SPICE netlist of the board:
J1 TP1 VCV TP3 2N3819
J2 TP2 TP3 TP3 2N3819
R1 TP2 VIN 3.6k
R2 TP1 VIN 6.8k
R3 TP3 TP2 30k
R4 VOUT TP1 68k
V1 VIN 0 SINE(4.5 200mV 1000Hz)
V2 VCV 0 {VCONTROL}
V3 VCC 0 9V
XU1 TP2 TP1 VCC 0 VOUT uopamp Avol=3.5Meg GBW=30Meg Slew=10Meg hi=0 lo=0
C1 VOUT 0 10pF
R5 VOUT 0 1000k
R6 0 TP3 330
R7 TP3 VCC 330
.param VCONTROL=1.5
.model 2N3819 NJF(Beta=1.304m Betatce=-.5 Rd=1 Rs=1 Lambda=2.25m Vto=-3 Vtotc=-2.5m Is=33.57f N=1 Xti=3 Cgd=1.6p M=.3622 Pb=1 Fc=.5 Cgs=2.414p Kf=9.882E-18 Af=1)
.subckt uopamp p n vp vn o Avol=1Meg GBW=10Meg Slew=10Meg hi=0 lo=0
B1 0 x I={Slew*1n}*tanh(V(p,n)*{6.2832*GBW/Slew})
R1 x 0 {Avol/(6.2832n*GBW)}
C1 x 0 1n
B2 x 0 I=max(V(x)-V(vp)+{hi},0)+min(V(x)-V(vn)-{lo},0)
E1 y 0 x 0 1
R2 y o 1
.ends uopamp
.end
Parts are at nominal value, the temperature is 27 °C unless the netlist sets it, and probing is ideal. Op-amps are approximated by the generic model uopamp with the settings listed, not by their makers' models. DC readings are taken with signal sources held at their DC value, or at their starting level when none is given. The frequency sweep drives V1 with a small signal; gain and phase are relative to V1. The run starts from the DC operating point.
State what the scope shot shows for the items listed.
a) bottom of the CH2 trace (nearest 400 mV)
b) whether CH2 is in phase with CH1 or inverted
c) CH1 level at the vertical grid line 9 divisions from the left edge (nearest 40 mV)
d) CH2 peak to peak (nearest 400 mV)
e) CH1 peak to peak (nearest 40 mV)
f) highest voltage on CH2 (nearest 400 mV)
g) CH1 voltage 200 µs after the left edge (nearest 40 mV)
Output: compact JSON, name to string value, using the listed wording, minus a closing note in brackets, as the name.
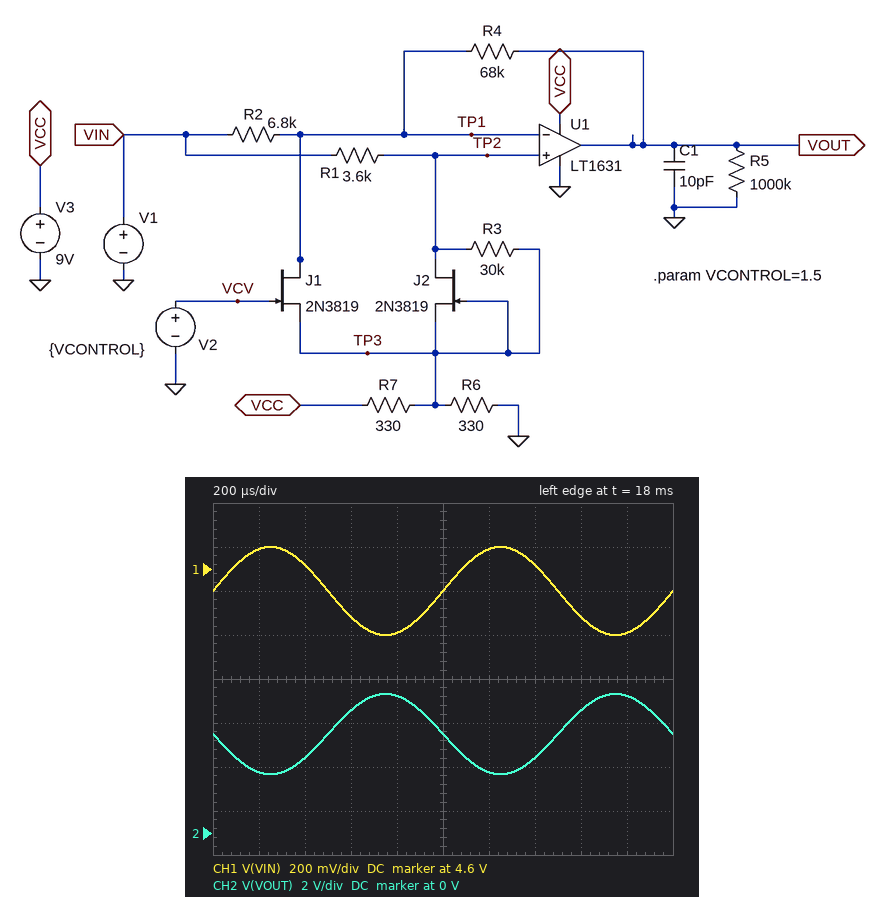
{"bottom of the CH2 trace": "2.8 V", "whether CH2 is in phase with CH1 or inverted": "inverted", "CH1 level at the vertical grid line 9 divisions from the left edge": "4.32 V", "CH2 peak to peak": "3.6 V", "CH1 peak to peak": "400 mV", "highest voltage on CH2": "6.4 V", "CH1 voltage 200 µs after the left edge": "4.68 V"}
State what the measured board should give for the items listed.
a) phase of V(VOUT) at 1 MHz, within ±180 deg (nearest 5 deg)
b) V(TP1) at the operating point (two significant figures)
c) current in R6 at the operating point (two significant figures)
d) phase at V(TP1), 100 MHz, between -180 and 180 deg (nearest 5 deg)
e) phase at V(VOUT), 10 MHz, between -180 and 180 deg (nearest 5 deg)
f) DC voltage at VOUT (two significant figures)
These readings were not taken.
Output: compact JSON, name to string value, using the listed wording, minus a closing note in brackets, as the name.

{"phase of V(VOUT) at 1 MHz, within ±180 deg": "160 deg", "V(TP1) at the operating point": "4.5 V", "current in R6 at the operating point": "14 mA", "phase at V(TP1), 100 MHz, between -180 and 180 deg": "-70 deg", "phase at V(VOUT), 10 MHz, between -180 and 180 deg": "85 deg", "DC voltage at VOUT": "4.5 V"}
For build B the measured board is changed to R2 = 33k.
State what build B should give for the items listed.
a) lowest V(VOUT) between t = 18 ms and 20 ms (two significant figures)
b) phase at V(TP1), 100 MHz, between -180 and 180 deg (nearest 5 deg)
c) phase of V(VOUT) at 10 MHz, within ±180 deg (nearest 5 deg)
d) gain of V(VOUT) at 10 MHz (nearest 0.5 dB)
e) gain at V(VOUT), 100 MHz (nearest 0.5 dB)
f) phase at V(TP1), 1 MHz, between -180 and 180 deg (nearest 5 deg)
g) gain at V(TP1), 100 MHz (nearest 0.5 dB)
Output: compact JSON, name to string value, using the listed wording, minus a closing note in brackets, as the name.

{"lowest V(VOUT) between t = 18 ms and 20 ms": "4.1 V", "phase at V(TP1), 100 MHz, between -180 and 180 deg": "-85 deg", "phase of V(VOUT) at 10 MHz, within ±180 deg": "75 deg", "gain of V(VOUT) at 10 MHz": "5.0 dB", "gain at V(VOUT), 100 MHz": "-31.5 dB", "phase at V(TP1), 1 MHz, between -180 and 180 deg": "35 deg", "gain at V(TP1), 100 MHz": "-24.5 dB"}
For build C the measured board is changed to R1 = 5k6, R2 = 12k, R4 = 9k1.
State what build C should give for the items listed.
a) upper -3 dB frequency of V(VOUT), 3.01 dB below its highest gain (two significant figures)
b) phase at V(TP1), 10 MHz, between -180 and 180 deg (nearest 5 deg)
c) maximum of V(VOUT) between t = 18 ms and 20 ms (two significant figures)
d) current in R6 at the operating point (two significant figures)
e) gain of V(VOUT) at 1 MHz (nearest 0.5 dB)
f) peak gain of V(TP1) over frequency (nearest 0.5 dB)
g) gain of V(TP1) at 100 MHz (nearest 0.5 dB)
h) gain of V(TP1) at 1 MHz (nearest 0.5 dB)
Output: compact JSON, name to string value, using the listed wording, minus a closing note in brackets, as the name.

{"upper -3 dB frequency of V(VOUT), 3.01 dB below its highest gain": "24 MHz", "phase at V(TP1), 10 MHz, between -180 and 180 deg": "45 deg", "maximum of V(VOUT) between t = 18 ms and 20 ms": "4.6 V", "current in R6 at the operating point": "14 mA", "gain of V(VOUT) at 1 MHz": "-3.5 dB", "peak gain of V(TP1) over frequency": "-7.5 dB", "gain of V(TP1) at 100 MHz": "-15.5 dB", "gain of V(TP1) at 1 MHz": "-25.0 dB"}
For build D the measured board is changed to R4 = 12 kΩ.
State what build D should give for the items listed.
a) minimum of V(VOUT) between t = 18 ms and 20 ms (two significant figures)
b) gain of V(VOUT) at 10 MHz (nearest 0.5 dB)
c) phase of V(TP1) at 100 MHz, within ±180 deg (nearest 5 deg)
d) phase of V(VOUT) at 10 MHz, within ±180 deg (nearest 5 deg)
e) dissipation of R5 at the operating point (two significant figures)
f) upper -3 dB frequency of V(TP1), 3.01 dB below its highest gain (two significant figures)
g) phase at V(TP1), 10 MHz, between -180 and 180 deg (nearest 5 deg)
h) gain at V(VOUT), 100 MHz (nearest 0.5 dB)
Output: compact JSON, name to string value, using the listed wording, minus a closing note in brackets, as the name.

{"minimum of V(VOUT) between t = 18 ms and 20 ms": "4.2 V", "gain of V(VOUT) at 10 MHz": "2.0 dB", "phase of V(TP1) at 100 MHz, within ±180 deg": "-65 deg", "phase of V(VOUT) at 10 MHz, within ±180 deg": "130 deg", "dissipation of R5 at the operating point": "20 µW", "upper -3 dB frequency of V(TP1), 3.01 dB below its highest gain": "55 MHz", "phase at V(TP1), 10 MHz, between -180 and 180 deg": "35 deg", "gain at V(VOUT), 100 MHz": "-22.5 dB"}
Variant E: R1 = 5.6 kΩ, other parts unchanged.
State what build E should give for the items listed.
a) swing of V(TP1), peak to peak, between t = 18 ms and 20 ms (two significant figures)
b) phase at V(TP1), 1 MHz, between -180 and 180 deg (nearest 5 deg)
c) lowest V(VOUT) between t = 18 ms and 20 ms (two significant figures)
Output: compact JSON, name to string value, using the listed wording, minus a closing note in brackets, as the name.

{"swing of V(TP1), peak to peak, between t = 18 ms and 20 ms": "20 mV", "phase at V(TP1), 1 MHz, between -180 and 180 deg": "60 deg", "lowest V(VOUT) between t = 18 ms and 20 ms": "2.6 V"}
